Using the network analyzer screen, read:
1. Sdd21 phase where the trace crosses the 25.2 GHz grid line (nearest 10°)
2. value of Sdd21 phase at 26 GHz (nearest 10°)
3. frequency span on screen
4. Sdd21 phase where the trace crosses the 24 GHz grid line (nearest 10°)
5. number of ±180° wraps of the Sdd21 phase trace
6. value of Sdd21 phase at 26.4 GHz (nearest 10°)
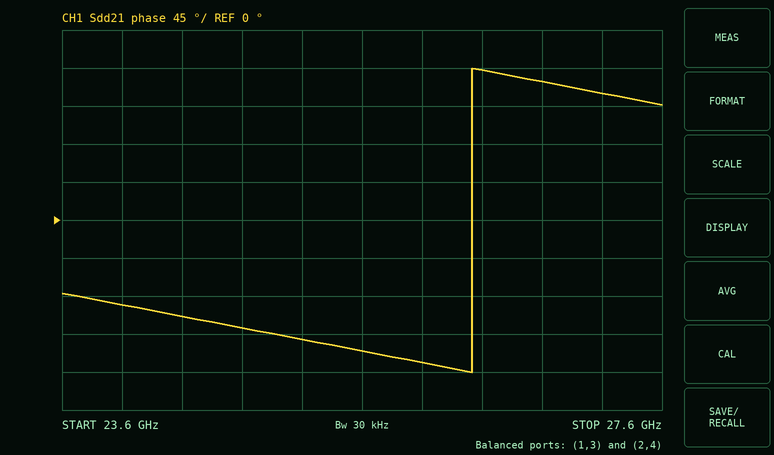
-140°
-170°
4 GHz
-100°
1
180°
